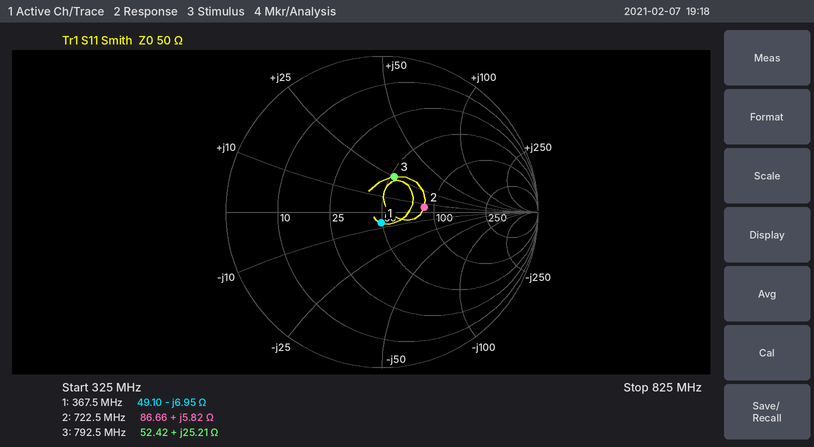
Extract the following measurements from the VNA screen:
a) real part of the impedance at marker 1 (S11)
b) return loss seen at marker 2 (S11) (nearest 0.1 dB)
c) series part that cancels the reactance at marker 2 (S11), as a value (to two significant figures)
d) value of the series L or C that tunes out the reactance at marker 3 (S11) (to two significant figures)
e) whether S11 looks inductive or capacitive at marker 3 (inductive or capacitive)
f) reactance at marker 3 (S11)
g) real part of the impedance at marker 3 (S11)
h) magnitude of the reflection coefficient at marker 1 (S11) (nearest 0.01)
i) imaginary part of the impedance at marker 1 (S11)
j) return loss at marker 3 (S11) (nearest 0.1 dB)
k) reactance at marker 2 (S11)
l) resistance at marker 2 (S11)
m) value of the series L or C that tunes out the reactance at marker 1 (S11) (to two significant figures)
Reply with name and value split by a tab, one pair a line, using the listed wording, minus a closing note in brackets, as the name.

real part of the impedance at marker 1	49.10 Ω
return loss seen at marker 2 (S11)	11.3 dB
series part that cancels the reactance at marker 2 (S11), as a value	38 pF
value of the series L or C that tunes out the reactance at marker 3 (S11)	8.0 pF
whether S11 looks inductive or capacitive at marker 3	inductive
reactance at marker 3	+25.21 Ω
real part of the impedance at marker 3	52.42 Ω
magnitude of the reflection coefficient at marker 1 (S11)	0.07
imaginary part of the impedance at marker 1	-6.95 Ω
return loss at marker 3 (S11)	12.4 dB
reactance at marker 2	+5.82 Ω
resistance at marker 2	86.66 Ω
value of the series L or C that tunes out the reactance at marker 1 (S11)	3.0 nH
